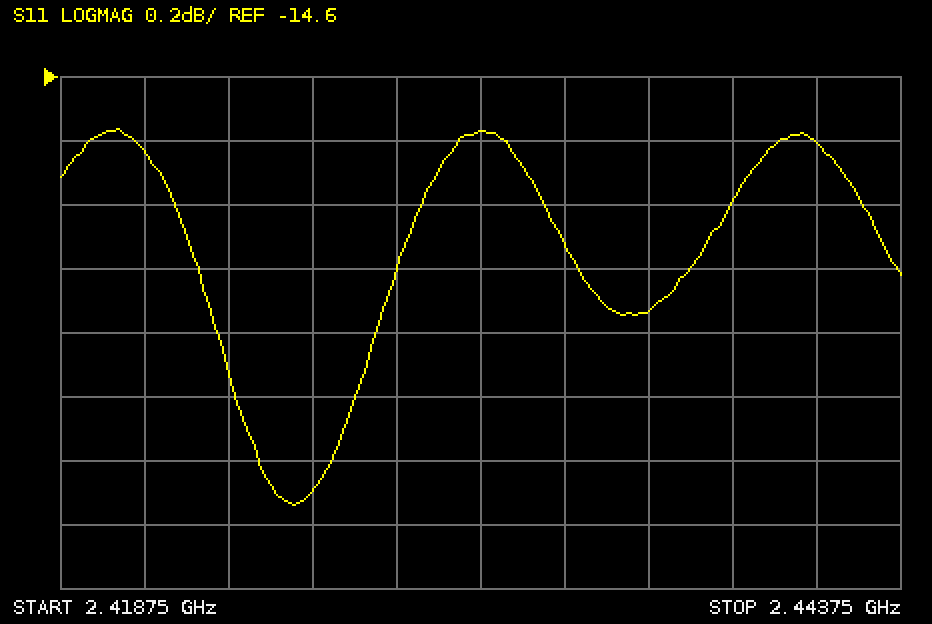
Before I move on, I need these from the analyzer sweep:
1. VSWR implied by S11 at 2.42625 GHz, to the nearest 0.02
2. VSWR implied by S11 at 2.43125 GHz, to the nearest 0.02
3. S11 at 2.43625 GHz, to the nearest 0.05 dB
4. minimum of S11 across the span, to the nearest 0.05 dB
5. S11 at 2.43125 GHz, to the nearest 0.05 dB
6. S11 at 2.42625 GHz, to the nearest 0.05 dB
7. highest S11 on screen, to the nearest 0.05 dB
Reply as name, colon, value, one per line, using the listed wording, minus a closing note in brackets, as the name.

VSWR implied by S11 at 2.42625 GHz, to the nearest 0.02: 1.38
VSWR implied by S11 at 2.43125 GHz, to the nearest 0.02: 1.44
S11 at 2.43625 GHz, to the nearest 0.05 dB: -15.35 dB
minimum of S11 across the span, to the nearest 0.05 dB: -15.95 dB
S11 at 2.43125 GHz, to the nearest 0.05 dB: -14.75 dB
S11 at 2.42625 GHz, to the nearest 0.05 dB: -15.90 dB
highest S11 on screen, to the nearest 0.05 dB: -14.75 dB
